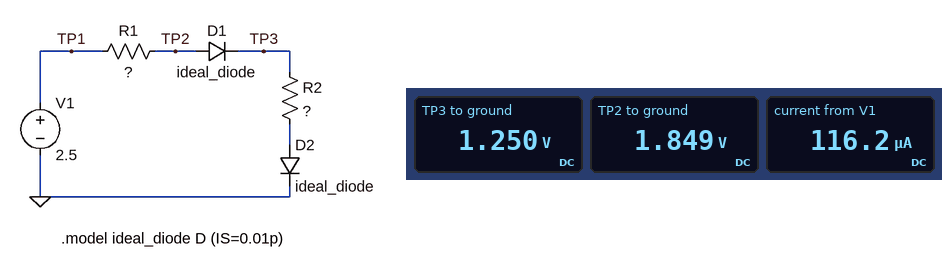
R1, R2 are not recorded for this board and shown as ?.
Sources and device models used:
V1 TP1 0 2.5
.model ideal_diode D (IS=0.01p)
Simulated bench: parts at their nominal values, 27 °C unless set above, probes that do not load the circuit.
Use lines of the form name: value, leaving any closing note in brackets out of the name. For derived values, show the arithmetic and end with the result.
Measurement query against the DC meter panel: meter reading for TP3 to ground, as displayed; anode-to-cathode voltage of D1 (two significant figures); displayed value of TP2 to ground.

meter reading for TP3 to ground, as displayed: 1.250 V
anode-to-cathode voltage of D1: 1.849 V - 1.25 V = 600 mV
displayed value of TP2 to ground: 1.849 V
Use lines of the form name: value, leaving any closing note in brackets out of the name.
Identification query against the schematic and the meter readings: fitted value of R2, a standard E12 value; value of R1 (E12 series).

fitted value of R2, a standard E12 value: 5.6 kΩ
value of R1: 5.6 kΩ
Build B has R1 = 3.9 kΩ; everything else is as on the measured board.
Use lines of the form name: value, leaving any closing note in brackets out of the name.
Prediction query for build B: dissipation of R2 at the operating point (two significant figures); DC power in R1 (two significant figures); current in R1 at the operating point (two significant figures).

dissipation of R2 at the operating point: 100 µW
DC power in R1: 72 µW
current in R1 at the operating point: 140 µA
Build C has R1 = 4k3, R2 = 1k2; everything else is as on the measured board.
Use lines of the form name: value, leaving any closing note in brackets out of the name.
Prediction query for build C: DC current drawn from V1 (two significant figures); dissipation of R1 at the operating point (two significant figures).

DC current drawn from V1: 230 µA
dissipation of R1 at the operating point: 230 µW
